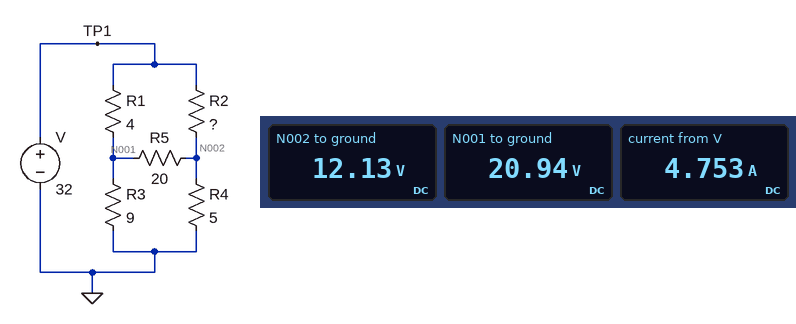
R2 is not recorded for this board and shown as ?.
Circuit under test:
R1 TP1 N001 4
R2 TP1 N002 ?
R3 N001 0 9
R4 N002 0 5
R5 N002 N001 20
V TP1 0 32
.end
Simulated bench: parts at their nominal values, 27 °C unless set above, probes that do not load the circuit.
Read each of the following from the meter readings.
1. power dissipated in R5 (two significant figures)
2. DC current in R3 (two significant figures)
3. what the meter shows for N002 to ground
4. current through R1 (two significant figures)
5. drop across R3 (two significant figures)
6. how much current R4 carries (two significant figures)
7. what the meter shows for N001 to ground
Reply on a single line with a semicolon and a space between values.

3.9 W; 2.3 A; 12.13 V; 2.8 A; 21 V; 2.4 A; 20.94 V
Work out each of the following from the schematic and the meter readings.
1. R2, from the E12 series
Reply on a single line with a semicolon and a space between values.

10 Ω
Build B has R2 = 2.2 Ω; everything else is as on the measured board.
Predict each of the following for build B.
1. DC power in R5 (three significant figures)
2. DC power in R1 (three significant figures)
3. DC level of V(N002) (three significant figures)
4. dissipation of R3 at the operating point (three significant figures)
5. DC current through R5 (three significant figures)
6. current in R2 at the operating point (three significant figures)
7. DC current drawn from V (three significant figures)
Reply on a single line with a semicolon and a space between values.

158 µW; 24.2 W; 22.2 V; 54.6 W; 2.81 mA; 4.45 A; 6.91 A
